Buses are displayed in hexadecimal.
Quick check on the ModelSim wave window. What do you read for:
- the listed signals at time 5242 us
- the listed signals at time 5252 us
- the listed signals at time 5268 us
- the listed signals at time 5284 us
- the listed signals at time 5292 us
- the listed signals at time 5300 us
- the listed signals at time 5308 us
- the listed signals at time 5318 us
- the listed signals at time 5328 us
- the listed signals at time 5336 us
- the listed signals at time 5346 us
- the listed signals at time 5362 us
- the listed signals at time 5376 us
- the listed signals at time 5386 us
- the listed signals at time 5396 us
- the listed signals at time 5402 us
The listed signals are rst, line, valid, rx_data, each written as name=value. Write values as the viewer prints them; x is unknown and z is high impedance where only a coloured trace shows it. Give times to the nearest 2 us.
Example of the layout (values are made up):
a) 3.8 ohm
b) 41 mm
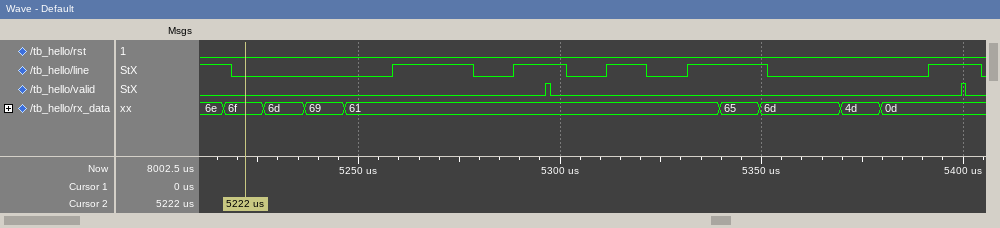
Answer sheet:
a) rst=0, line=0, valid=0, rx_data=69
b) rst=0, line=0, valid=0, rx_data=61
c) rst=0, line=1, valid=0, rx_data=61
d) rst=0, line=0, valid=0, rx_data=61
e) rst=0, line=1, valid=0, rx_data=61
f) rst=0, line=1, valid=0, rx_data=61
g) rst=0, line=0, valid=0, rx_data=61
h) rst=0, line=1, valid=0, rx_data=61
i) rst=0, line=0, valid=0, rx_data=61
j) rst=0, line=1, valid=0, rx_data=61
k) rst=0, line=1, valid=0, rx_data=65
l) rst=0, line=0, valid=0, rx_data=6d
m) rst=0, line=0, valid=0, rx_data=4d
n) rst=0, line=0, valid=0, rx_data=0d
o) rst=0, line=1, valid=0, rx_data=0d
p) rst=0, line=1, valid=0, rx_data=0d
